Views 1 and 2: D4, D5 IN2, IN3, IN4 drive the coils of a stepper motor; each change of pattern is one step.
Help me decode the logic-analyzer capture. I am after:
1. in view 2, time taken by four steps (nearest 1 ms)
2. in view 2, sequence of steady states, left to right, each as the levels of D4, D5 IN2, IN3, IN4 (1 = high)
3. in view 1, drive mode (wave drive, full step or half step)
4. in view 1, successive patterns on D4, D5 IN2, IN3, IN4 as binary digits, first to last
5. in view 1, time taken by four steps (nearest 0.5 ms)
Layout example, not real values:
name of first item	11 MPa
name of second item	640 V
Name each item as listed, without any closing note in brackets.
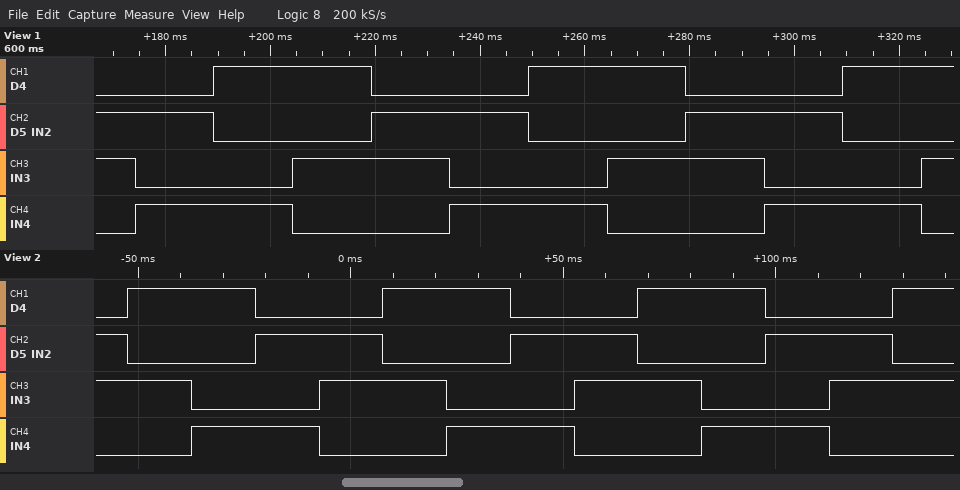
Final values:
in view 2, time taken by four steps	60 ms
in view 2, sequence of steady states, left to right, each as the levels of D4, D5 IN2, IN3, IN4	0110 1010 1001 0101 0110 1010 1001 0101 0110 1010 1001 0101 0110 1010
in view 1, drive mode	full step
in view 1, successive patterns on D4, D5 IN2, IN3, IN4 as binary digits, first to last	0110 0101 1001 1010 0110 0101 1001 1010 0110 0101 1001 1010
in view 1, time taken by four steps	60.0 ms
